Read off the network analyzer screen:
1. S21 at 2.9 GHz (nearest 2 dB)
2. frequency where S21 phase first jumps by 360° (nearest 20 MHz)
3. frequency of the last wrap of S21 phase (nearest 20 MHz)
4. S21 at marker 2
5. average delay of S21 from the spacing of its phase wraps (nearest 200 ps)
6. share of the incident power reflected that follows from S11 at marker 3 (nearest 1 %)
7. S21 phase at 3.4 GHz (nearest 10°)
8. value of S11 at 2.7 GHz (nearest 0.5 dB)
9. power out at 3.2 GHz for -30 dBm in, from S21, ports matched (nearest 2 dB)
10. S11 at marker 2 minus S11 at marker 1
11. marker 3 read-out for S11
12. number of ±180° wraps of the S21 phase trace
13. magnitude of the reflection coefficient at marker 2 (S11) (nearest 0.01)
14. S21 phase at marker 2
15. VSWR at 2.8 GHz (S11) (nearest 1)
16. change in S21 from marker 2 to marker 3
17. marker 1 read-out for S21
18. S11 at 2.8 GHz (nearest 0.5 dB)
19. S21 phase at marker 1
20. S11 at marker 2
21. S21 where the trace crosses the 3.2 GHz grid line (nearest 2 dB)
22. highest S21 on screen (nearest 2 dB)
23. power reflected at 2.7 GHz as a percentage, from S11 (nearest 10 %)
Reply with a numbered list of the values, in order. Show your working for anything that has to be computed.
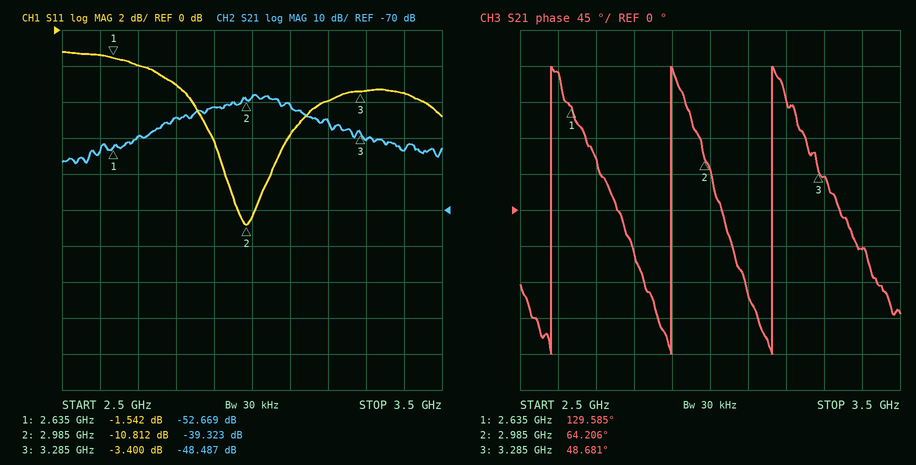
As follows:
1. -42 dB
2. 2.58 GHz
3. 3.16 GHz
4. -39.323 dB
5. 2 cycles / (3.16 GHz − 2.58 GHz) ≈ 3.4 ns
6. 10^(-3.4/10) ≈ 46 %
7. -50°
8. -2.0 dB
9. -30 dBm + (-46 dB) = -76 dBm
10. -10.812 − (-1.542) = -9.270 dB
11. -3.400 dB
12. 3
13. 10^(-10.812/20) ≈ 0.29
14. 64.206°
15. |Γ| = 10^(-3/20) = 0.7079; VSWR = (1 + 0.7079)/(1 − 0.7079) ≈ 6
16. -48.487 − (-39.323) = -9.164 dB
17. -52.669 dB
18. -3.0 dB
19. 129.585°
20. -10.812 dB
21. -46 dB
22. -38 dB
23. 10^(-2/10) ≈ 63.1 %, so 60 % to the nearest 10 %
